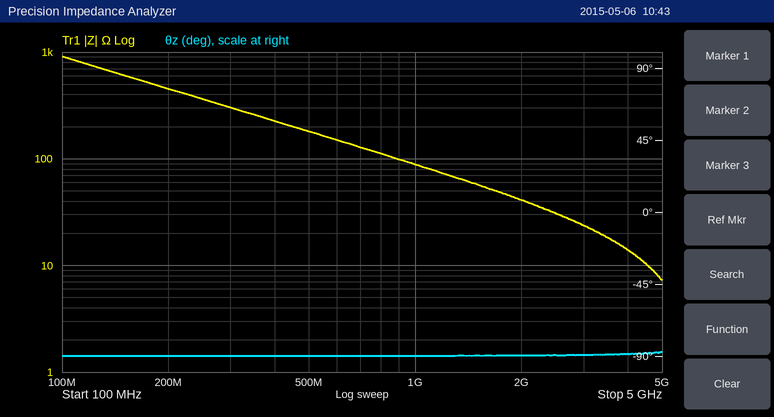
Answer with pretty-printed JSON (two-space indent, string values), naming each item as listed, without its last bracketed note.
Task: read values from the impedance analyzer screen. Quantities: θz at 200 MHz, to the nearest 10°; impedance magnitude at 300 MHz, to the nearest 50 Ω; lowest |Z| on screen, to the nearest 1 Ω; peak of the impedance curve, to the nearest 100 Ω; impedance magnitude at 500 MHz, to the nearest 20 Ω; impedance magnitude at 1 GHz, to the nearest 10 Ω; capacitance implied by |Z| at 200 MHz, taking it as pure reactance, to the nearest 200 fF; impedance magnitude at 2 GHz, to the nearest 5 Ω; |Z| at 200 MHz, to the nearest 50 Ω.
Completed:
{
  "θz at 200 MHz, to the nearest 10°": "-90°",
  "impedance magnitude at 300 MHz, to the nearest 50 Ω": "300 Ω",
  "lowest |Z| on screen, to the nearest 1 Ω": "7 Ω",
  "peak of the impedance curve, to the nearest 100 Ω": "900 Ω",
  "impedance magnitude at 500 MHz, to the nearest 20 Ω": "180 Ω",
  "impedance magnitude at 1 GHz, to the nearest 10 Ω": "90 Ω",
  "capacitance implied by |Z| at 200 MHz, taking it as pure reactance, to the nearest 200 fF": "1.8 pF",
  "impedance magnitude at 2 GHz, to the nearest 5 Ω": "40 Ω",
  "|Z| at 200 MHz, to the nearest 50 Ω": "450 Ω"
}
